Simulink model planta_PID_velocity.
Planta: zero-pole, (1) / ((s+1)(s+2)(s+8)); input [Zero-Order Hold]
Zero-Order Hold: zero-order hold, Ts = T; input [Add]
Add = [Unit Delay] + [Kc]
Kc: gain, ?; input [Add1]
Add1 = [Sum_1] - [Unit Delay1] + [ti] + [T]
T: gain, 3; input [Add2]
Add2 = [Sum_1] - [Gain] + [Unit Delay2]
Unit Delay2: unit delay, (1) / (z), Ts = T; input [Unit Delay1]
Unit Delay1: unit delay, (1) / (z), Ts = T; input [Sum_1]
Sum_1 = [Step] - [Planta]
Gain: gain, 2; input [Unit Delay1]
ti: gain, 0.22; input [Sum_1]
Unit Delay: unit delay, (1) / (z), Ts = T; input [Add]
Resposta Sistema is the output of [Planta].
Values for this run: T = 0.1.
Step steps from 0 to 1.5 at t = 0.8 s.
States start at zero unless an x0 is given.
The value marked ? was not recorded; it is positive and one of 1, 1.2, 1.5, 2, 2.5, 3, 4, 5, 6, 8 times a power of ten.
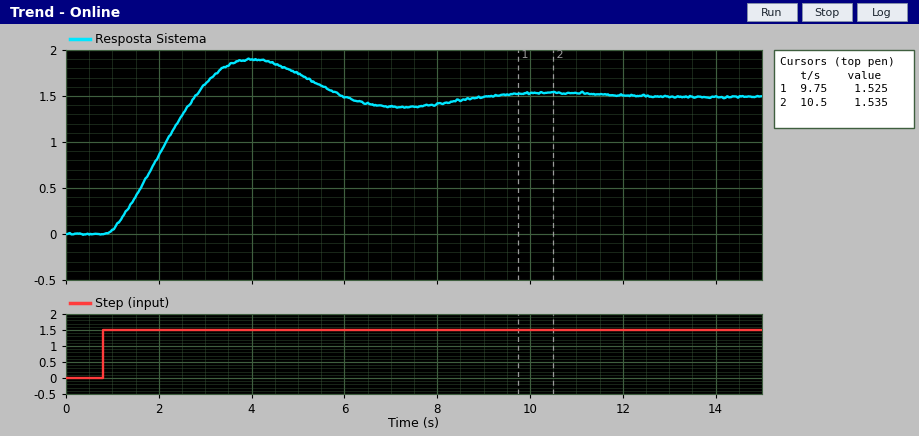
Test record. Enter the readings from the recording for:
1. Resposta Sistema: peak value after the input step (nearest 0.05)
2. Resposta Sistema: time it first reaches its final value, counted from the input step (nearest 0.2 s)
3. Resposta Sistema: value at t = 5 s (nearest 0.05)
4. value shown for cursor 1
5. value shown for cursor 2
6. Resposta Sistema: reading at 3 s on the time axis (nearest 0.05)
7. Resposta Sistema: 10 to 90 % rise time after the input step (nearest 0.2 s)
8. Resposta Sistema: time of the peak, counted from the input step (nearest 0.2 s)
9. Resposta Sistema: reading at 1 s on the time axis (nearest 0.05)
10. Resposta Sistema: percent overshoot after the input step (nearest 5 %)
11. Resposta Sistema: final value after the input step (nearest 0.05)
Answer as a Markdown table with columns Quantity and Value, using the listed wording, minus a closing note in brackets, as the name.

| Quantity | Value |
|---|---|
| Resposta Sistema: peak value after the input step | 1.90 |
| Resposta Sistema: time it first reaches its final value, counted from the input step | 2.0 s |
| Resposta Sistema: value at t = 5 s | 1.75 |
| value shown for cursor 1 | 1.525 |
| value shown for cursor 2 | 1.535 |
| Resposta Sistema: reading at 3 s on the time axis | 1.65 |
| Resposta Sistema: 10 to 90 % rise time after the input step | 1.4 s |
| Resposta Sistema: time of the peak, counted from the input step | 3.2 s |
| Resposta Sistema: reading at 1 s on the time axis | 0.05 |
| Resposta Sistema: percent overshoot after the input step | 25 % |
| Resposta Sistema: final value after the input step | 1.50 |
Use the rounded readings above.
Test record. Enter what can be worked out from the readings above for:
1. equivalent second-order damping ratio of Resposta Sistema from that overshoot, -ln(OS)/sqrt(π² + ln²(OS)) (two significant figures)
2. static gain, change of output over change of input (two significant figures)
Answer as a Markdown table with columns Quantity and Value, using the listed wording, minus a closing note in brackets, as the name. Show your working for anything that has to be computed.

| Quantity | Value |
|---|---|
| equivalent second-order damping ratio of Resposta Sistema from that overshoot, -ln(OS)/sqrt(π² + ln²(OS)) | ln(0.25) = -1.386; 1.386 / sqrt(9.870 + 1.922) = 0.40 |
| static gain, change of output over change of input | (1.5 - 0) / (1.5 - 0) = 1.0 |
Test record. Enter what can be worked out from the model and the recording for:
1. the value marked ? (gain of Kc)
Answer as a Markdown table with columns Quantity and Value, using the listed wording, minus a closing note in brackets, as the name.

| Quantity | Value |
|---|---|
| the value marked ? | 10 |
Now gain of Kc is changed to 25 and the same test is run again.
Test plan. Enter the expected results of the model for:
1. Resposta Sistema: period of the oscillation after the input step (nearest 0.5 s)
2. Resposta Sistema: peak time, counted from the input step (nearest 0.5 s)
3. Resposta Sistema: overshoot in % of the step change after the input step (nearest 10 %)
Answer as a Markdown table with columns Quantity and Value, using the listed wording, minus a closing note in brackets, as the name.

| Quantity | Value |
|---|---|
| Resposta Sistema: period of the oscillation after the input step | 4.0 s |
| Resposta Sistema: peak time, counted from the input step | 2.0 s |
| Resposta Sistema: overshoot in % of the step change after the input step | 40 % |
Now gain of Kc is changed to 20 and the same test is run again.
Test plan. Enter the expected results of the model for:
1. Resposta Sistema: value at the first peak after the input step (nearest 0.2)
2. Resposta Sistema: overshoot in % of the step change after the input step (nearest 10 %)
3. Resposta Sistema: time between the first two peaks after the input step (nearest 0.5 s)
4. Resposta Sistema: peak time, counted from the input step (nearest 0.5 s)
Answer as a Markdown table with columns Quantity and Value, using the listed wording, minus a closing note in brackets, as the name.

| Quantity | Value |
|---|---|
| Resposta Sistema: value at the first peak after the input step | 2.0 |
| Resposta Sistema: overshoot in % of the step change after the input step | 40 % |
| Resposta Sistema: time between the first two peaks after the input step | 4.5 s |
| Resposta Sistema: peak time, counted from the input step | 2.0 s |
